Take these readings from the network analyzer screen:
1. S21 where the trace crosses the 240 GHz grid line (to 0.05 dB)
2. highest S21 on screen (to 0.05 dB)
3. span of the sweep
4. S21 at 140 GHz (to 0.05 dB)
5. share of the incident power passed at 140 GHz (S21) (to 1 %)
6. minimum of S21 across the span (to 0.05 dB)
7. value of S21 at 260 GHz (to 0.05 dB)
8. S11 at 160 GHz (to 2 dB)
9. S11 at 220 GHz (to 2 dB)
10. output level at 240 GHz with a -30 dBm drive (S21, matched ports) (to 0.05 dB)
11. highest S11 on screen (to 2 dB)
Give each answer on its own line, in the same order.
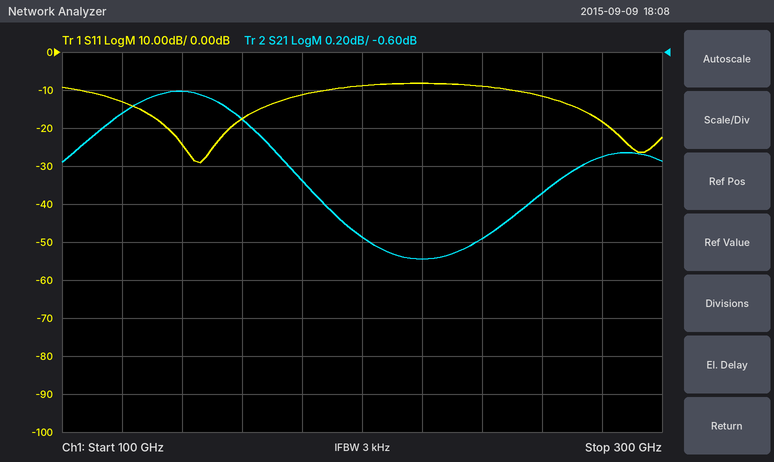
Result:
-1.60 dB
-0.80 dB
200 GHz
-0.80 dB
83 %
-1.70 dB
-1.35 dB
-18 dB
-8 dB
-31.60 dBm
-8 dB
